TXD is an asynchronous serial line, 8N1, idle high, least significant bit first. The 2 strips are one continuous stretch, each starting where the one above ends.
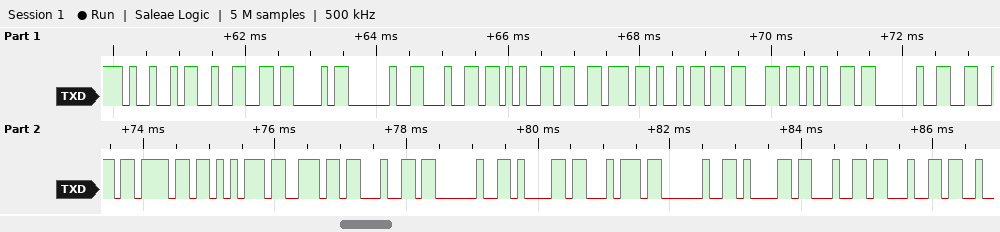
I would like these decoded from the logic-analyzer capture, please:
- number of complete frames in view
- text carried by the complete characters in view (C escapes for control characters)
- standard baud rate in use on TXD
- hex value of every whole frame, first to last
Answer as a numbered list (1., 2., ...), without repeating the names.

1. 23
2. "I2C device found at add"
3. 9600 baud
4. 49 32 43 20 64 65 76 69 63 65 20 66 6F 75 6E 64 20 61 74 20 61 64 64
